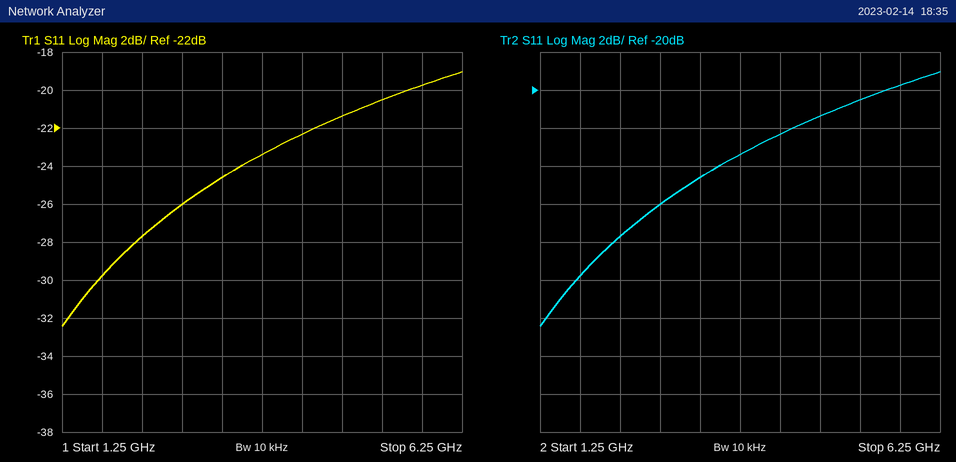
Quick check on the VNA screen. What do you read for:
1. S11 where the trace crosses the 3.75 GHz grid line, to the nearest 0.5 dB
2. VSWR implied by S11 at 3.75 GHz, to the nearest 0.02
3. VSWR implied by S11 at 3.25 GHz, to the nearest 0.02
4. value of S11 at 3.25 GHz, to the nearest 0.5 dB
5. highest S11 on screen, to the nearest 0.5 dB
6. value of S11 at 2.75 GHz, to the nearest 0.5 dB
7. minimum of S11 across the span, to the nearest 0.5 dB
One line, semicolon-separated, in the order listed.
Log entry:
-23.5 dB; 1.14; 1.12; -24.5 dB; -19.0 dB; -26.0 dB; -32.5 dB
